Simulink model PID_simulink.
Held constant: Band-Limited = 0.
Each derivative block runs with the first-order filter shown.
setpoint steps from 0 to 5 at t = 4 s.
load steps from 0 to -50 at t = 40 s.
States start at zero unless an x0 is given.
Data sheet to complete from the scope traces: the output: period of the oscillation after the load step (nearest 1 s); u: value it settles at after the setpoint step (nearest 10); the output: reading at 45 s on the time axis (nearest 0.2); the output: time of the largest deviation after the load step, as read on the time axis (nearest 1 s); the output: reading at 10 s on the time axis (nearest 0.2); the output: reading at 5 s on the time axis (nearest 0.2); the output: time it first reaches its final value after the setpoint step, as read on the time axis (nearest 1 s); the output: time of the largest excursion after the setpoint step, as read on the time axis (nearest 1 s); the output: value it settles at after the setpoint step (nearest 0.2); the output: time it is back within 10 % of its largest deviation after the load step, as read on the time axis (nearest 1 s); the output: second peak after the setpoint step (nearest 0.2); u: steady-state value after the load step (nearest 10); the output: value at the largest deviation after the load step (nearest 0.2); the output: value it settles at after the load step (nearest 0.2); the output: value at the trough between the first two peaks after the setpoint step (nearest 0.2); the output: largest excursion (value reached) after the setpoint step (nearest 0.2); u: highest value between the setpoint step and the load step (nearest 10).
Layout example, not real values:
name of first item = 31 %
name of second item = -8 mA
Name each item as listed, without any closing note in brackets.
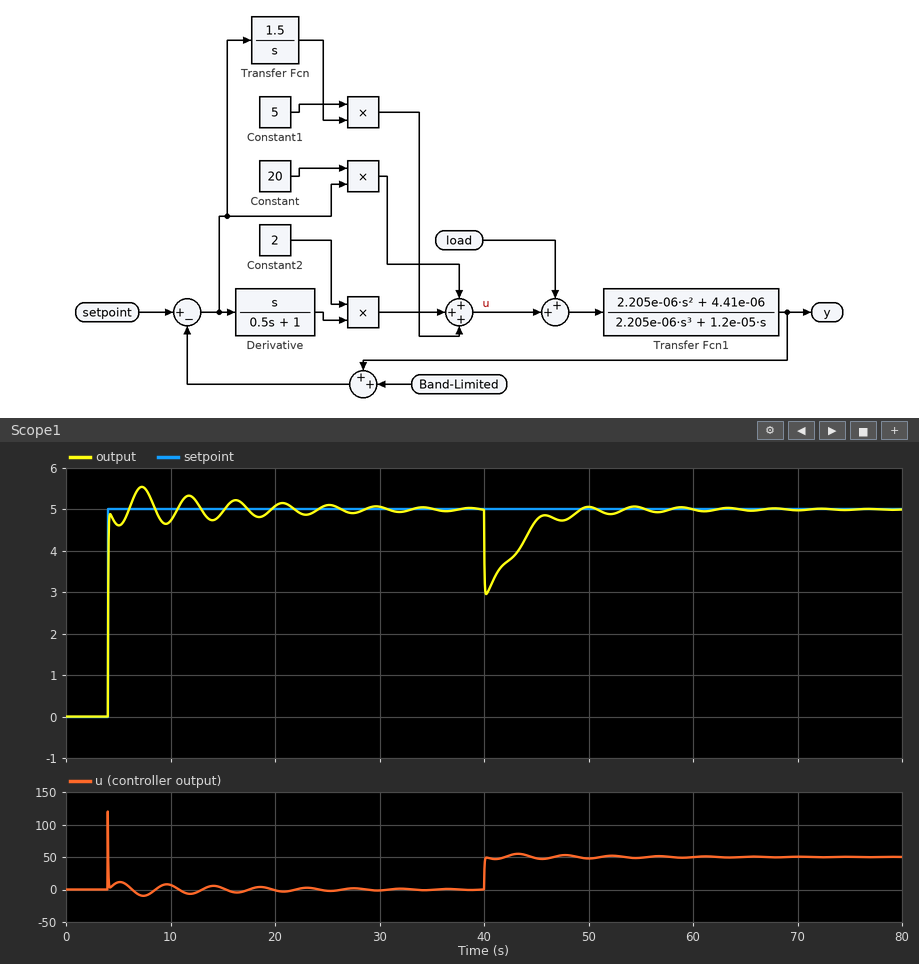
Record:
the output: period of the oscillation after the load step = 12 s
u: value it settles at after the setpoint step = 0
the output: reading at 45 s on the time axis = 4.8
the output: time of the largest deviation after the load step, as read on the time axis = 40 s
the output: reading at 10 s on the time axis = 4.8
the output: reading at 5 s on the time axis = 4.6
the output: time it first reaches its final value after the setpoint step, as read on the time axis = 6 s
the output: time of the largest excursion after the setpoint step, as read on the time axis = 7 s
the output: value it settles at after the setpoint step = 5.0
the output: time it is back within 10 % of its largest deviation after the load step, as read on the time axis = 48 s
the output: second peak after the setpoint step = 5.4
u: steady-state value after the load step = 50
the output: value at the largest deviation after the load step = 3.0
the output: value it settles at after the load step = 5.0
the output: value at the trough between the first two peaks after the setpoint step = 4.6
the output: largest excursion (value reached) after the setpoint step = 5.6
u: highest value between the setpoint step and the load step = 120
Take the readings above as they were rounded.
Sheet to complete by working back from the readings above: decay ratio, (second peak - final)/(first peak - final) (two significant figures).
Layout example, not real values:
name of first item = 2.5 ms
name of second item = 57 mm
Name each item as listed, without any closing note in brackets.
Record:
decay ratio, (second peak - final)/(first peak - final) = 0.67
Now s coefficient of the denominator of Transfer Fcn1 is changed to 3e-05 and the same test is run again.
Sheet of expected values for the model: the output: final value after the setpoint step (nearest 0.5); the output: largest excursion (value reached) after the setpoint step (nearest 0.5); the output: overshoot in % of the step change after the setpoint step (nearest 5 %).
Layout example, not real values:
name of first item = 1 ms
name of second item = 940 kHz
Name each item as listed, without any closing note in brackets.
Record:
the output: final value after the setpoint step = 5.0
the output: largest excursion (value reached) after the setpoint step = 6.0
the output: overshoot in % of the step change after the setpoint step = 25 %
